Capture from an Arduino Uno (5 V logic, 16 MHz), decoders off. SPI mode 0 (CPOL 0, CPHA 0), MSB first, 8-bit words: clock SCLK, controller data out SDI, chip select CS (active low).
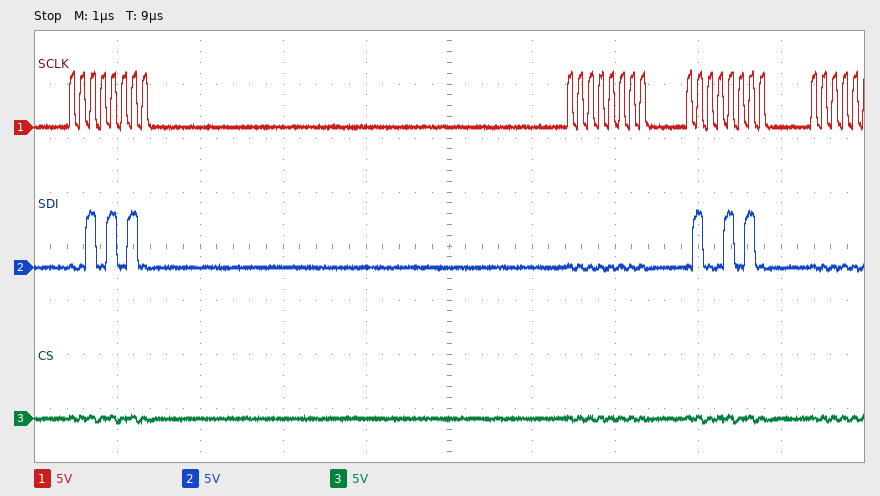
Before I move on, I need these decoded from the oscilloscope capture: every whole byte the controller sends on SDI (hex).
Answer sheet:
2A 00 4A
